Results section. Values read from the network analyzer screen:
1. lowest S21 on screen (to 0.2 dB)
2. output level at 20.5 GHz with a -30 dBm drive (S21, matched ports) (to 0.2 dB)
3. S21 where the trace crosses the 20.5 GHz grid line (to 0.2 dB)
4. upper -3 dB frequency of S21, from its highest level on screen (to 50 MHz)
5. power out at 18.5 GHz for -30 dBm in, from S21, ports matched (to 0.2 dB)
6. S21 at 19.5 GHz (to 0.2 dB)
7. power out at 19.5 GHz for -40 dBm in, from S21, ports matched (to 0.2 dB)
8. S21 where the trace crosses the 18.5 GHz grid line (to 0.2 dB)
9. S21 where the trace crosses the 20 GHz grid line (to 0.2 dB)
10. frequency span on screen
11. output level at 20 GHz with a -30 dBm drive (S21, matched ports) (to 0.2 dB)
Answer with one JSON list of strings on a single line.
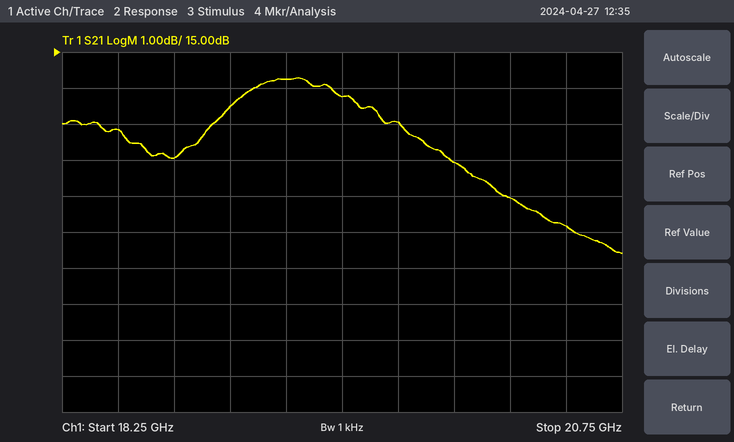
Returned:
["9.4 dB", "-19.8 dBm", "10.2 dB", "20.15 GHz", "-17.2 dBm", "13.8 dB", "-26.2 dBm", "12.8 dB", "12.0 dB", "2.5 GHz", "-18.0 dBm"]
